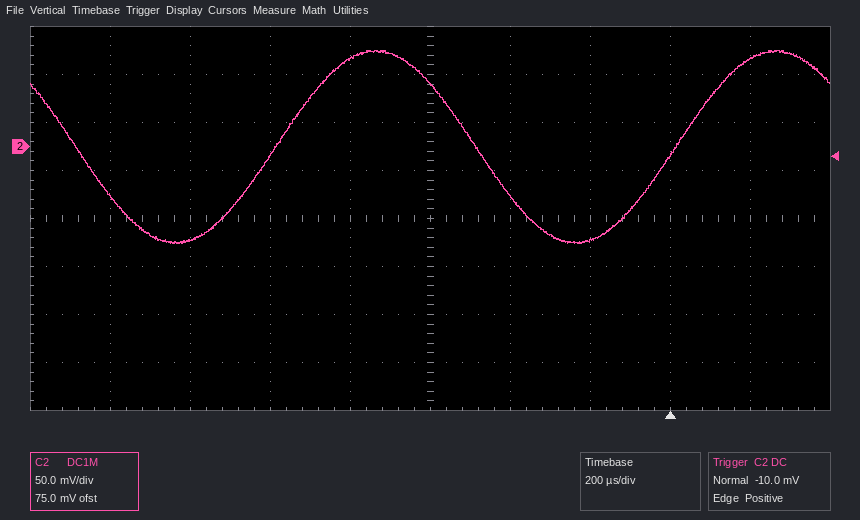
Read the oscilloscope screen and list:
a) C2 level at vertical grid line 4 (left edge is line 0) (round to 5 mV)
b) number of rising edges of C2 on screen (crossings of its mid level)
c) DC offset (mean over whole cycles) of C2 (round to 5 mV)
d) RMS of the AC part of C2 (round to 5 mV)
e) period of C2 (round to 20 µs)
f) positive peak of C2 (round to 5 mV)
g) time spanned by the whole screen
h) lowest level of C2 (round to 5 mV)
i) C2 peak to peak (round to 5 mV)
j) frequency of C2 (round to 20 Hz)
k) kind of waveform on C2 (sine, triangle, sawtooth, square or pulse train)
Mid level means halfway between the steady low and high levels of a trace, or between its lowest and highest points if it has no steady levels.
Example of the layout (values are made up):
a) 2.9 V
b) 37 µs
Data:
a) 90 mV
b) 2
c) 0 mV
d) 70 mV
e) 1.00 ms
f) 100 mV
g) 2 ms
h) -100 mV
i) 200 mV
j) 1.00 kHz
k) sine
